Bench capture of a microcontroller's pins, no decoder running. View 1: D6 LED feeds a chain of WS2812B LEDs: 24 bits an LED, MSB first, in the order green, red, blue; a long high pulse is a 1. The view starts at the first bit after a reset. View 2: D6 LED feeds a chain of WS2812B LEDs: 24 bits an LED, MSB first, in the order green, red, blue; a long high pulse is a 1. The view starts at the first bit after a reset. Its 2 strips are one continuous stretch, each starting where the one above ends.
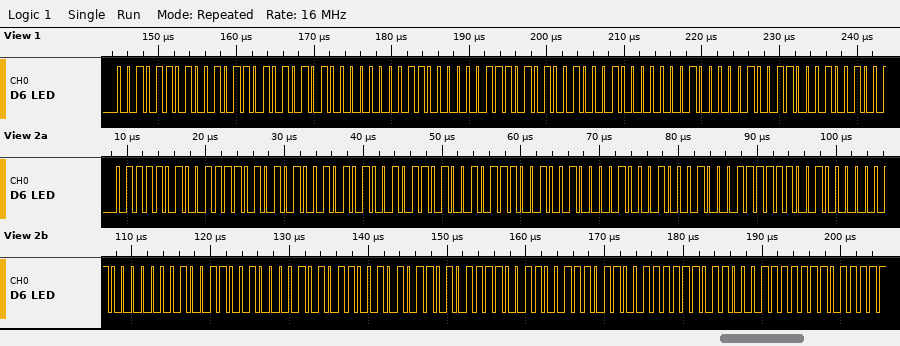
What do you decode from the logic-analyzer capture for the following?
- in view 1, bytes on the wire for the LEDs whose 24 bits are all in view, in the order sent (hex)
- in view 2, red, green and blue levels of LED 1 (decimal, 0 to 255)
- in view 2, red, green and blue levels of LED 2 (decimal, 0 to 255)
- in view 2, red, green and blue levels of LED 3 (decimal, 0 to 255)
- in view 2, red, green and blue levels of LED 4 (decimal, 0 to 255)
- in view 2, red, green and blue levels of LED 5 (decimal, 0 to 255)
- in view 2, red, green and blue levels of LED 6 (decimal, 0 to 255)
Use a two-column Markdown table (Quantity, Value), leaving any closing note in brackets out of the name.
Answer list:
| Quantity | Value |
|---|---|
| in view 1, bytes on the wire for the LEDs whose 24 bits are all in view, in the order sent | 2D 2D 54 03 03 A9 10 10 4C |
| in view 2, red, green and blue levels of LED 1 | 122, 122, 165 |
| in view 2, red, green and blue levels of LED 2 | 75, 75, 146 |
| in view 2, red, green and blue levels of LED 3 | 17, 17, 249 |
| in view 2, red, green and blue levels of LED 4 | 2, 2, 100 |
| in view 2, red, green and blue levels of LED 5 | 43, 43, 94 |
| in view 2, red, green and blue levels of LED 6 | 103, 103, 236 |
